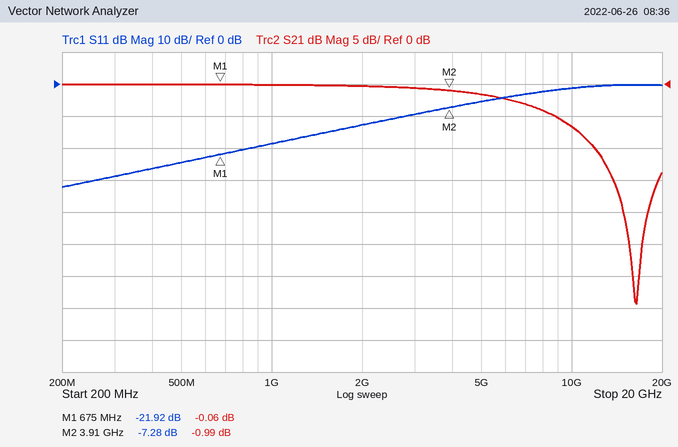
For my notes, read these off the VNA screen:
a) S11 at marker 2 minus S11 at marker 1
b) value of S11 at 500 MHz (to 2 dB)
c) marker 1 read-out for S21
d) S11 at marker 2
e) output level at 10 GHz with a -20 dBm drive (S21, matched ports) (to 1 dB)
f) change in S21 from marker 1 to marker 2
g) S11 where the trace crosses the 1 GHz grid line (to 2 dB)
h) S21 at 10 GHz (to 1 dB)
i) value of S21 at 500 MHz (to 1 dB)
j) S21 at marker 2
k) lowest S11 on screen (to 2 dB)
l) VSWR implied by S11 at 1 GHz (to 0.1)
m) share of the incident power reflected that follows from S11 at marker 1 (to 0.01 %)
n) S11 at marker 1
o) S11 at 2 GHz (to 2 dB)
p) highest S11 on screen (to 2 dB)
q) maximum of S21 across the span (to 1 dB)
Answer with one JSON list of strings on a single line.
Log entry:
["14.64 dB", "-24 dB", "-0.06 dB", "-7.28 dB", "-27 dBm", "-0.93 dB", "-18 dB", "-7 dB", "0 dB", "-0.99 dB", "-32 dB", "1.3", "0.64 %", "-21.92 dB", "-12 dB", "0 dB", "0 dB"]
